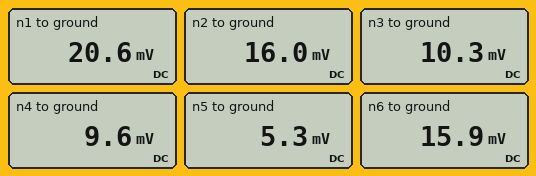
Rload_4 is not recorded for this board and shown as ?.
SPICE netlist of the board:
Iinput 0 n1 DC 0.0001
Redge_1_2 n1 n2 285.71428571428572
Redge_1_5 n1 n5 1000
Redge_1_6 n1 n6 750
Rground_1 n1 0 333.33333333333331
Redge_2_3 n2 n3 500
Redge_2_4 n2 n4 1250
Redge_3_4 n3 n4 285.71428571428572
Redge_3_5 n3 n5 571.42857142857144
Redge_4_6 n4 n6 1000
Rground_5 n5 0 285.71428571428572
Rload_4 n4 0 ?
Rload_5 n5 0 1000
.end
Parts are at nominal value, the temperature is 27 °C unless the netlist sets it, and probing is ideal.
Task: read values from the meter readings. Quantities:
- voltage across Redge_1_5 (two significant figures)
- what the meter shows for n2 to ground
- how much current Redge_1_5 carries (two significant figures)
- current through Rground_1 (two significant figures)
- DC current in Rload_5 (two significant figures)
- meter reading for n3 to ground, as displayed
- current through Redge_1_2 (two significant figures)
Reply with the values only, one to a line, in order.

15 mV
16.0 mV
15 µA
62 µA
5.3 µA
10.3 mV
16 µA
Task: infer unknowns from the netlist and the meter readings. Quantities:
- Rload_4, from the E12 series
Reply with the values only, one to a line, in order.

680 Ω
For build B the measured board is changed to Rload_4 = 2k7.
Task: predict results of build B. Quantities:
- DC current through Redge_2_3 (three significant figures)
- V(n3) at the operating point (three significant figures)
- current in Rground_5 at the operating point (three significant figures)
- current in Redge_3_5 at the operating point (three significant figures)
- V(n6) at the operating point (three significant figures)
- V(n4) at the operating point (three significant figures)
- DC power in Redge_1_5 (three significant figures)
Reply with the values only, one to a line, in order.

9.86 µA
13.4 mV
22.0 µA
12.5 µA
18.7 mV
14.2 mV
251 nW
